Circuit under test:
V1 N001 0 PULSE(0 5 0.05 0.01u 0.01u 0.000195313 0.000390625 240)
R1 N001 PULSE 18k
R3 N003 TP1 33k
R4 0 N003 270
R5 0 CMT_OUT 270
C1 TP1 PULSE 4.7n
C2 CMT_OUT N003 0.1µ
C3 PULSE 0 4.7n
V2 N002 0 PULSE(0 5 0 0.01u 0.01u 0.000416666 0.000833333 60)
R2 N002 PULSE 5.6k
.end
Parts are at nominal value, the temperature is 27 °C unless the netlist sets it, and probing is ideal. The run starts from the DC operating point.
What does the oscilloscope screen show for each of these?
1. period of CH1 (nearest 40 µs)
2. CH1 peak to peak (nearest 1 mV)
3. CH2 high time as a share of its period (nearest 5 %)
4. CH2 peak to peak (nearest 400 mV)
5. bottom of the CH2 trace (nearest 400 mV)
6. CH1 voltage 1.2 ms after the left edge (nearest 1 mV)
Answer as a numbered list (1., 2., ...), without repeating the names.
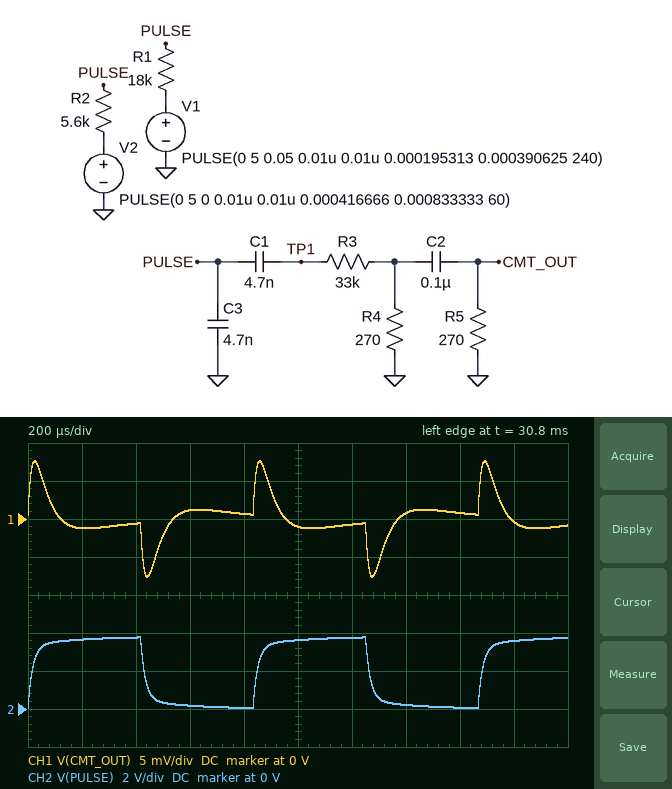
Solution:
1. 840 µs
2. 15 mV
3. 50 %
4. 3.6 V
5. 0 V
6. -1 mV
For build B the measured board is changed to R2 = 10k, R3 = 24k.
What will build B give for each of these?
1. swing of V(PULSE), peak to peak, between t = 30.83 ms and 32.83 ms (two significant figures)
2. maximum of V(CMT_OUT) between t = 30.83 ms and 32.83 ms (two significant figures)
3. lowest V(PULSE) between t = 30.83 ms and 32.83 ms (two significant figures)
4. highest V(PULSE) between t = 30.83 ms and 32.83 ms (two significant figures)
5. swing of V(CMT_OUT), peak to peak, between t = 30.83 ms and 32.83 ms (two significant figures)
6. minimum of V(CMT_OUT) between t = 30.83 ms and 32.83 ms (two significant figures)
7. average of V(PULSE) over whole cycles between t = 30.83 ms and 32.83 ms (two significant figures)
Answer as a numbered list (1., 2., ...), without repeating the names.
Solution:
1. 3.1 V
2. 6.7 mV
3. 57 mV
4. 3.2 V
5. 13 mV
6. -6.7 mV
7. 1.6 V
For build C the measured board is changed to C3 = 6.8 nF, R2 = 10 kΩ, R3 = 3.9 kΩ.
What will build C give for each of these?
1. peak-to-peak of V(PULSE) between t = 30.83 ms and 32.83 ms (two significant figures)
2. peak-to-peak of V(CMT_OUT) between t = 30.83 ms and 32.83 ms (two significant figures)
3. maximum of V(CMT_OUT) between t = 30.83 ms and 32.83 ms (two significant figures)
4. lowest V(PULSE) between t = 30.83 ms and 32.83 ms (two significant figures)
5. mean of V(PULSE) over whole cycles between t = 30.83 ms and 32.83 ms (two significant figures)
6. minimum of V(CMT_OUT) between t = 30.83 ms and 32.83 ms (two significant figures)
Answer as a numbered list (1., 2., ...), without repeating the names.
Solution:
1. 3.2 V
2. 29 mV
3. 15 mV
4. 19 mV
5. 1.6 V
6. -15 mV
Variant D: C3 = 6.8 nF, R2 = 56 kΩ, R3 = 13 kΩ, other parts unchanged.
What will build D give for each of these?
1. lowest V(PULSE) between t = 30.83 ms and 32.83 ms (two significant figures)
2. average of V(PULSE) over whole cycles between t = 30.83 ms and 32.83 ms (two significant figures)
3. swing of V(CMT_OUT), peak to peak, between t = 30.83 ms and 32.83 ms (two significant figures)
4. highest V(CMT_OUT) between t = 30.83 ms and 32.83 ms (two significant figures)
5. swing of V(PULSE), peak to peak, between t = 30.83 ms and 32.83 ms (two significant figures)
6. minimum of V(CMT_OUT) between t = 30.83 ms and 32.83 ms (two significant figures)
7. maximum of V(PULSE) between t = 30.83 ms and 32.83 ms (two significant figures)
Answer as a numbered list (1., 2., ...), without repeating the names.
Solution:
1. 96 mV
2. 610 mV
3. 3.7 mV
4. 1.9 mV
5. 1.0 V
6. -1.9 mV
7. 1.1 V
